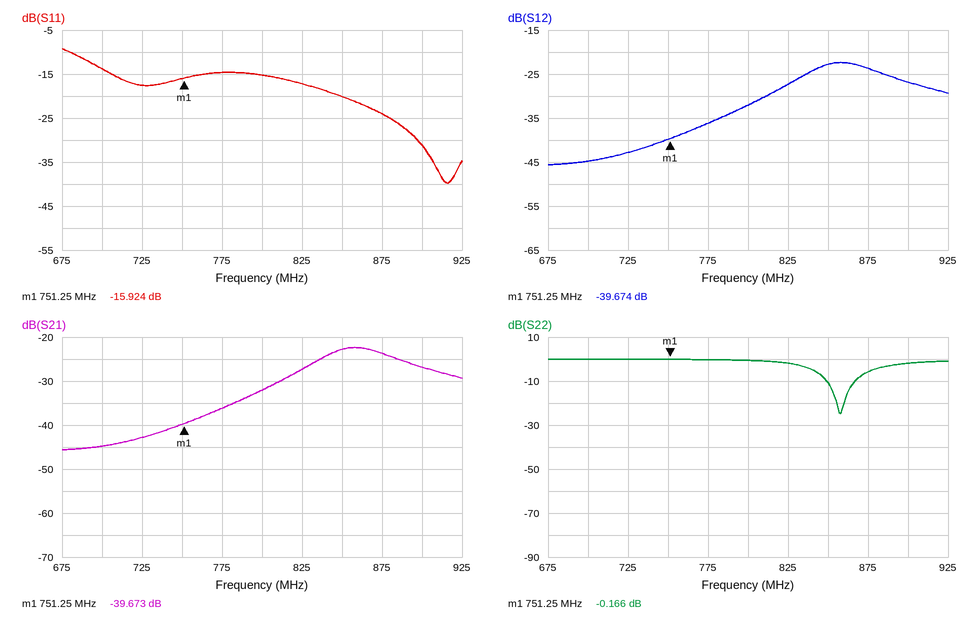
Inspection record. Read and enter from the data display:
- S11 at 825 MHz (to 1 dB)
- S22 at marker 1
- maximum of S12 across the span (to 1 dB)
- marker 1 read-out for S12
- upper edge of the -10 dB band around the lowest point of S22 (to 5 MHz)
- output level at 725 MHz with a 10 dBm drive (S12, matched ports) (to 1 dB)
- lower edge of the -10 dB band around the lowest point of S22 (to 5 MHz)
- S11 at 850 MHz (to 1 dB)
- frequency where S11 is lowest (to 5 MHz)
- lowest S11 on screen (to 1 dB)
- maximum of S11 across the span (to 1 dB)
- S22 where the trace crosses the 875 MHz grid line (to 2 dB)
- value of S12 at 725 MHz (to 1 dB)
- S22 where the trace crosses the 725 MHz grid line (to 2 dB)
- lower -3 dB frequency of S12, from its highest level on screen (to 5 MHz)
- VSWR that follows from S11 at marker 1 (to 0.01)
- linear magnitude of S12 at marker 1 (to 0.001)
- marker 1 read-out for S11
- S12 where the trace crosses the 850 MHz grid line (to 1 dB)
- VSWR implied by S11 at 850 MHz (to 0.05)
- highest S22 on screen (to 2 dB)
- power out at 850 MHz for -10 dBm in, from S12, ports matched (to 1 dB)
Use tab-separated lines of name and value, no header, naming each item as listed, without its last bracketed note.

S11 at 825 MHz	-17 dB
S22 at marker 1	-0.166 dB
maximum of S12 across the span	-22 dB
marker 1 read-out for S12	-39.674 dB
upper edge of the -10 dB band around the lowest point of S22	865 MHz
output level at 725 MHz with a 10 dBm drive (S12, matched ports)	-33 dBm
lower edge of the -10 dB band around the lowest point of S22	850 MHz
S11 at 850 MHz	-20 dB
frequency where S11 is lowest	915 MHz
lowest S11 on screen	-40 dB
maximum of S11 across the span	-9 dB
S22 where the trace crosses the 875 MHz grid line	-6 dB
value of S12 at 725 MHz	-43 dB
S22 where the trace crosses the 725 MHz grid line	0 dB
lower -3 dB frequency of S12, from its highest level on screen	835 MHz
VSWR that follows from S11 at marker 1	1.38
linear magnitude of S12 at marker 1	0.010
marker 1 read-out for S11	-15.924 dB
S12 where the trace crosses the 850 MHz grid line	-23 dB
VSWR implied by S11 at 850 MHz	1.20
highest S22 on screen	0 dB
power out at 850 MHz for -10 dBm in, from S12, ports matched	-33 dBm
